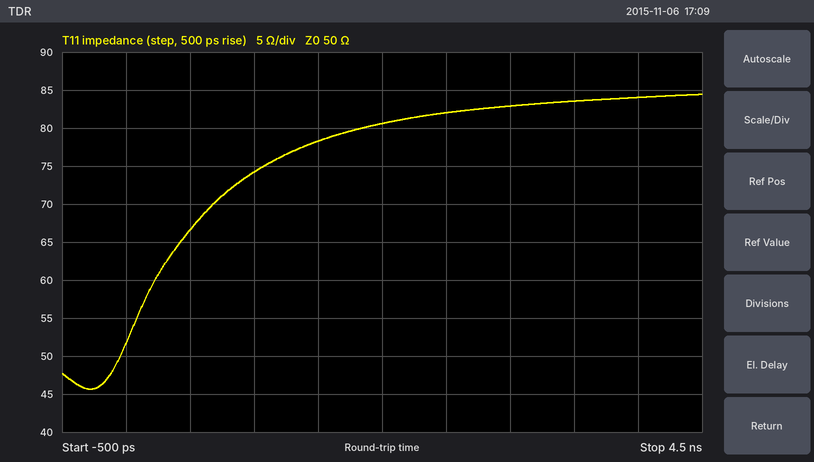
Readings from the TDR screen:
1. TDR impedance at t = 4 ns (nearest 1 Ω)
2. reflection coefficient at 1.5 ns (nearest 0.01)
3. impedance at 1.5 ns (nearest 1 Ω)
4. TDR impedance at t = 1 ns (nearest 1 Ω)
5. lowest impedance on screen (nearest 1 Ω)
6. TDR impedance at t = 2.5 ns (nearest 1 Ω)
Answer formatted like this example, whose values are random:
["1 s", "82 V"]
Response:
["84 Ω", "+0.22", "78 Ω", "74 Ω", "46 Ω", "82 Ω"]
